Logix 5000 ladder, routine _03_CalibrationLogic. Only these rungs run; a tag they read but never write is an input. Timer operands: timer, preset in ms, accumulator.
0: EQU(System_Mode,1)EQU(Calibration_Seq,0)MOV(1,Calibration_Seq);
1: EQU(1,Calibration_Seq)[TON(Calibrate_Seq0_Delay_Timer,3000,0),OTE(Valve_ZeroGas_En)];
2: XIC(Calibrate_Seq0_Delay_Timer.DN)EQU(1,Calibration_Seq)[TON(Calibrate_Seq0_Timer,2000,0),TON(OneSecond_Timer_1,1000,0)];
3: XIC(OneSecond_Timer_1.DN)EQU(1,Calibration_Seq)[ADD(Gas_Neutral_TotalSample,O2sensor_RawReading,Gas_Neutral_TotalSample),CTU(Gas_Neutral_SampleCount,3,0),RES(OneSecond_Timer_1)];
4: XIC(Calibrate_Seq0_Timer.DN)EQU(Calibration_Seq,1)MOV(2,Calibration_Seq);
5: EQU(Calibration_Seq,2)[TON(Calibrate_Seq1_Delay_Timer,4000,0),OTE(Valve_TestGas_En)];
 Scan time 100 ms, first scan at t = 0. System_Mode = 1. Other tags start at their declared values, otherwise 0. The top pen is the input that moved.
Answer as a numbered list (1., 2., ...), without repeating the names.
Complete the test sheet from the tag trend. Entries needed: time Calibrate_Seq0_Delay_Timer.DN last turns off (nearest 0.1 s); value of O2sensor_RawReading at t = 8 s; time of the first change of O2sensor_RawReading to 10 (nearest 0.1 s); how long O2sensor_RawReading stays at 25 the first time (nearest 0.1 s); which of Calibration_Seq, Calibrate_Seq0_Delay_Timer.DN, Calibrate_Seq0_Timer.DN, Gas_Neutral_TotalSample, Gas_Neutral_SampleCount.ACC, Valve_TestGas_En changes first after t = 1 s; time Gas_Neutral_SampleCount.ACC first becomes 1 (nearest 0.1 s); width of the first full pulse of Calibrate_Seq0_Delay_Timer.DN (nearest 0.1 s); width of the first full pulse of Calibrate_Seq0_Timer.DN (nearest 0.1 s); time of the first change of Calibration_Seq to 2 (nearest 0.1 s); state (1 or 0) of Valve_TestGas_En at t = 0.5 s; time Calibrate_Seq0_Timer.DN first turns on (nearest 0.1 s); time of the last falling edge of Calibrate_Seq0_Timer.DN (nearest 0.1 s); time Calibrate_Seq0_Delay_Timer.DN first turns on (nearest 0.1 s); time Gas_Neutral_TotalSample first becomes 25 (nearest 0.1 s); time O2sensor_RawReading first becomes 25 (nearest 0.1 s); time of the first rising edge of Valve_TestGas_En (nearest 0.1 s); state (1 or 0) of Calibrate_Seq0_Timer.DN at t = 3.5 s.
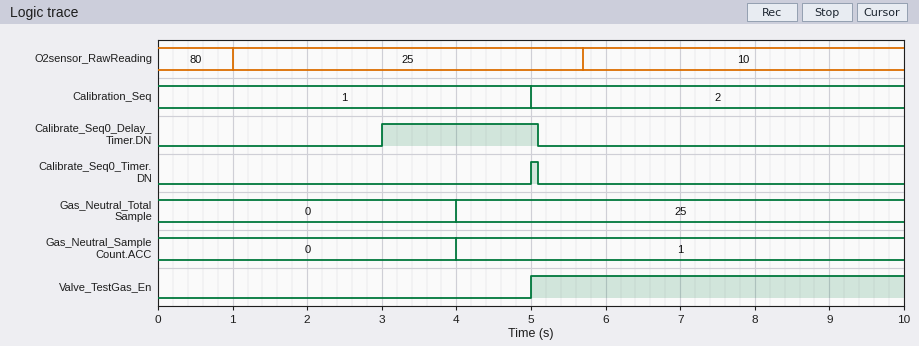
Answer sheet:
1. 5.1 s
2. 10
3. 5.7 s
4. 4.7 s
5. Calibrate_Seq0_Delay_Timer.DN
6. 4.0 s
7. 2.1 s
8. 0.1 s
9. 5.0 s
10. 0
11. 5.0 s
12. 5.1 s
13. 3.0 s
14. 4.0 s
15. 1.0 s
16. 5.0 s
17. 0
